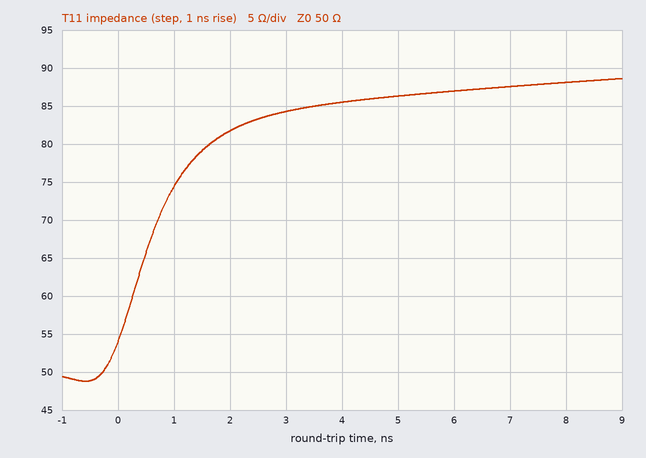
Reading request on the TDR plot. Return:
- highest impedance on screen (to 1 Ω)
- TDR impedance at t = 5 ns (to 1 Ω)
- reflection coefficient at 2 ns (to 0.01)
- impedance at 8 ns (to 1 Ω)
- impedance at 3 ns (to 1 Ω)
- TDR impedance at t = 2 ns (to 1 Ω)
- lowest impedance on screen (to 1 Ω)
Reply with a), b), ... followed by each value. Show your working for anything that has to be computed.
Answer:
a) 89 Ω
b) 86 Ω
c) (82 − 50)/(82 + 50) ≈ +0.24
d) 88 Ω
e) 84 Ω
f) 82 Ω
g) 49 Ω
